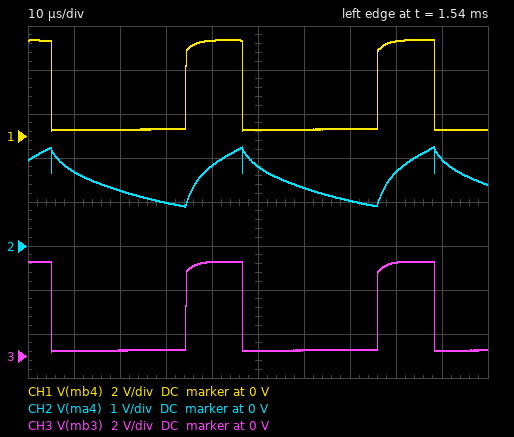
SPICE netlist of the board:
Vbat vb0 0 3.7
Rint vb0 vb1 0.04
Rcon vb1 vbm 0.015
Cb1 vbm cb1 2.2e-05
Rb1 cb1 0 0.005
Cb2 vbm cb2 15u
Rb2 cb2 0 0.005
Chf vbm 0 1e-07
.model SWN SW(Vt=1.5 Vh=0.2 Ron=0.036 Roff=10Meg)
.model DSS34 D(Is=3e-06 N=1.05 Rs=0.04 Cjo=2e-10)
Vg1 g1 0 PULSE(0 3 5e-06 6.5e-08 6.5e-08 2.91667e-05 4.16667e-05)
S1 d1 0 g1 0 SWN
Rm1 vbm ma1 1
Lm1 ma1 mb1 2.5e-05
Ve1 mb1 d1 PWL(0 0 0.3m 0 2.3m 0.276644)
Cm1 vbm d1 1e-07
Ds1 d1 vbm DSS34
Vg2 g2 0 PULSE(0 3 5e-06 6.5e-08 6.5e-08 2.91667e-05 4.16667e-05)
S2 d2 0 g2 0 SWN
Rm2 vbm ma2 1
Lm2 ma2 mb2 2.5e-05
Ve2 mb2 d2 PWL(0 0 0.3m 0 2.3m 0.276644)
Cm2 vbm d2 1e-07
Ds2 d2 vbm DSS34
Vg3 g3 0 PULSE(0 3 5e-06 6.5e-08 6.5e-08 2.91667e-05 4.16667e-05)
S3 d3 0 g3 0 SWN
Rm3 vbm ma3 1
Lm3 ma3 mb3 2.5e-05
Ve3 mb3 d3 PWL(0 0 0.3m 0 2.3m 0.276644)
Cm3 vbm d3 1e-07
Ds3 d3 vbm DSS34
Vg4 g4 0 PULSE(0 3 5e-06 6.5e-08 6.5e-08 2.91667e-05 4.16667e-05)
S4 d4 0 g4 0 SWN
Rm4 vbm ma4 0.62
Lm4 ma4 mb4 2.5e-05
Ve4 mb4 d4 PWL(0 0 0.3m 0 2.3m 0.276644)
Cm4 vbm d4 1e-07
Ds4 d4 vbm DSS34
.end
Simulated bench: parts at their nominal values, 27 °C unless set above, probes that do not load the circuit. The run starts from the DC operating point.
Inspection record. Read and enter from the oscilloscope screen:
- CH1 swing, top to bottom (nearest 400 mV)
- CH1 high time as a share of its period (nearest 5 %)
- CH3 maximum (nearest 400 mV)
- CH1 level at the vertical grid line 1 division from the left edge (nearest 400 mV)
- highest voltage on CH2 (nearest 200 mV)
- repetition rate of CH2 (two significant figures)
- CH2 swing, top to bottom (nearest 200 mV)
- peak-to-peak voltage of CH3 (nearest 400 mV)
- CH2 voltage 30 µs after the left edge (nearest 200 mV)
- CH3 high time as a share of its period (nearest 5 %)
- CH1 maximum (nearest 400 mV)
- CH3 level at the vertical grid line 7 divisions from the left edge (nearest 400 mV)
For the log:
4.0 V
30 %
4.4 V
400 mV
2.2 V
24 kHz
1.4 V
4.0 V
1.0 V
30 %
4.4 V
400 mV
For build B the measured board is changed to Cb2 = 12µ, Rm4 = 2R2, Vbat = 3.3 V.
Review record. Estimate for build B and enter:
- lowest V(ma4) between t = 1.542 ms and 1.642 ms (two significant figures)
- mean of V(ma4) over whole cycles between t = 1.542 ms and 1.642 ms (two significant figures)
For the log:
330 mV
1.3 V
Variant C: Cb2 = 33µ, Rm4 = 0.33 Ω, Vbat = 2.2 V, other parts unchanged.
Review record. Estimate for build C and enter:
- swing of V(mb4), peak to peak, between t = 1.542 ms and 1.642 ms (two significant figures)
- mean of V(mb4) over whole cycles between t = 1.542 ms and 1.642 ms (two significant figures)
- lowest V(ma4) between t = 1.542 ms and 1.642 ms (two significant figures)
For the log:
2.6 V
1.0 V
740 mV
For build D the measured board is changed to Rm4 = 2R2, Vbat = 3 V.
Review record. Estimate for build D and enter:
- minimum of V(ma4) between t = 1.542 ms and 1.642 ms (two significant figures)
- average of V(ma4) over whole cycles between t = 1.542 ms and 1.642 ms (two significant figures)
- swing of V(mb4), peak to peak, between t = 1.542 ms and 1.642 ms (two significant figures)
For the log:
320 mV
1.2 V
3.3 V
